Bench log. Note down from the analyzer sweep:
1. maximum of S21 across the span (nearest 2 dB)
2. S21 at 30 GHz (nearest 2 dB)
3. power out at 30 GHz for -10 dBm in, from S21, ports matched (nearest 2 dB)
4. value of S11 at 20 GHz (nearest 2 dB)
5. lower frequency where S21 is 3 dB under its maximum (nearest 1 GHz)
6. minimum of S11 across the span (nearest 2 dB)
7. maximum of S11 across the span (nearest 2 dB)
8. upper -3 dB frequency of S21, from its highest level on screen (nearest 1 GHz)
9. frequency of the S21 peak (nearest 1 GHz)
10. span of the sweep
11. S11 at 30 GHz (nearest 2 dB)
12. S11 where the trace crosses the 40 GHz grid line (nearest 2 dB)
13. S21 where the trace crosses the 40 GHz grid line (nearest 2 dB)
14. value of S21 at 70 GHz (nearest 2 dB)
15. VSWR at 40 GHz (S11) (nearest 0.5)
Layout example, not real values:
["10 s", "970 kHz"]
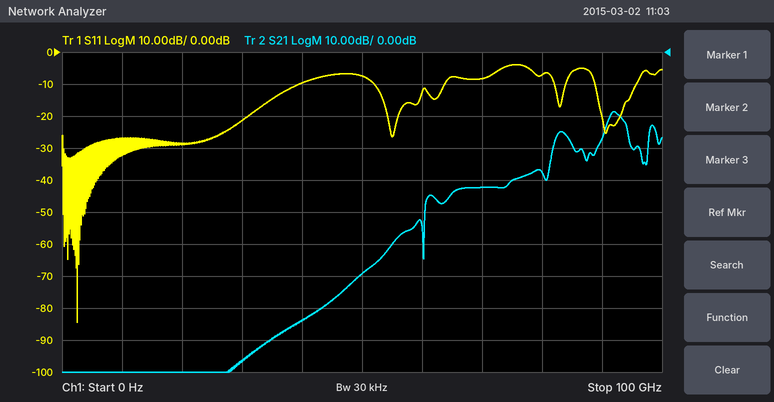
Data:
["-18 dB", "-96 dB", "-106 dBm", "-28 dB", "91 GHz", "-84 dB", "-4 dB", "94 GHz", "92 GHz", "100 GHz", "-22 dB", "-10 dB", "-84 dB", "-42 dB", "2.0"]
